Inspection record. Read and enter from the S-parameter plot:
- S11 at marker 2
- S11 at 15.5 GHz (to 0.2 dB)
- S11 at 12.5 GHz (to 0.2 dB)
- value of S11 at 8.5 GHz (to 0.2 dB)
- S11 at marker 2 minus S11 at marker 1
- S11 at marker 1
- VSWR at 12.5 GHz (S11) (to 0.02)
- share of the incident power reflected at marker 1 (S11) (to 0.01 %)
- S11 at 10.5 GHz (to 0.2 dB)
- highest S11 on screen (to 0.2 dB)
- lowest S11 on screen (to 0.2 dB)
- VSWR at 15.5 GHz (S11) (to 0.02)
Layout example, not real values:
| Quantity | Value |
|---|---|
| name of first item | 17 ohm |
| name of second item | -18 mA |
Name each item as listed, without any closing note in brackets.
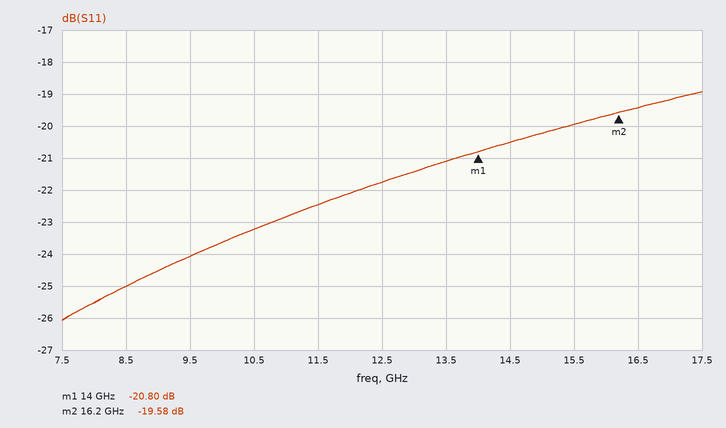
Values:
| Quantity | Value |
|---|---|
| S11 at marker 2 | -19.58 dB |
| S11 at 15.5 GHz | -20.0 dB |
| S11 at 12.5 GHz | -21.8 dB |
| value of S11 at 8.5 GHz | -25.0 dB |
| S11 at marker 2 minus S11 at marker 1 | 1.22 dB |
| S11 at marker 1 | -20.80 dB |
| VSWR at 12.5 GHz (S11) | 1.18 |
| share of the incident power reflected at marker 1 (S11) | 0.83 % |
| S11 at 10.5 GHz | -23.2 dB |
| highest S11 on screen | -19.0 dB |
| lowest S11 on screen | -26.0 dB |
| VSWR at 15.5 GHz (S11) | 1.22 |
